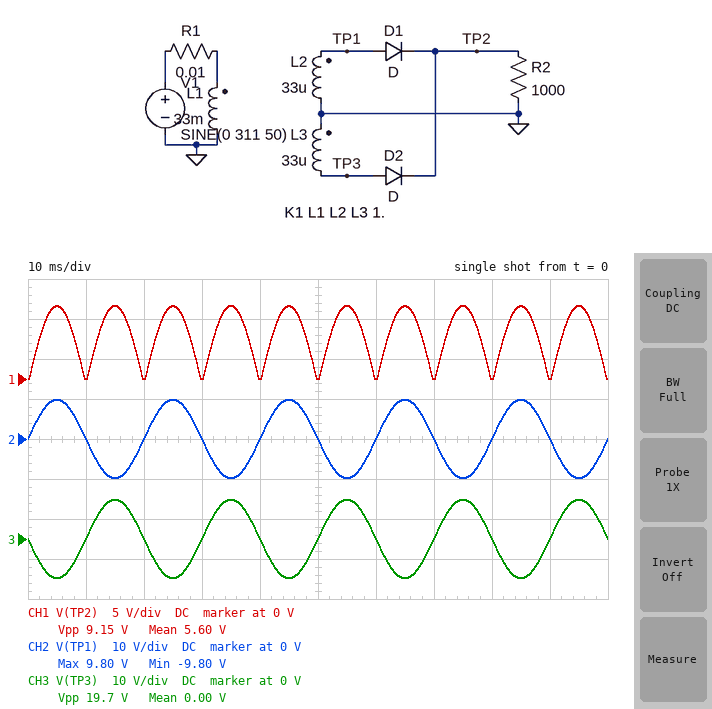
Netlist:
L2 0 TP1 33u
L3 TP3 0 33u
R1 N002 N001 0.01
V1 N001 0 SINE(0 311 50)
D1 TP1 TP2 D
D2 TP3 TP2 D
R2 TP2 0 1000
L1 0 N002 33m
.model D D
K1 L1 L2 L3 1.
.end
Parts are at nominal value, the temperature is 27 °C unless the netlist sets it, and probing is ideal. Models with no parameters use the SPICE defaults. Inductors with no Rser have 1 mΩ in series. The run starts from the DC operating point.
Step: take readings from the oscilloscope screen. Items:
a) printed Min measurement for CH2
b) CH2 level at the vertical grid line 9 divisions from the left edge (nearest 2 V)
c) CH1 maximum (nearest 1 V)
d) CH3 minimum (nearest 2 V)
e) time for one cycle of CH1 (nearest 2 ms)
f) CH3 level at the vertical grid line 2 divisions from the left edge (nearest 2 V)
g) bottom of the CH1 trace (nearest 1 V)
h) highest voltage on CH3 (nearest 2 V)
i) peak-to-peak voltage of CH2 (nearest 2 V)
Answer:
-9.80 V
0 V
9 V
-10 V
10 ms
0 V
0 V
10 V
20 V
